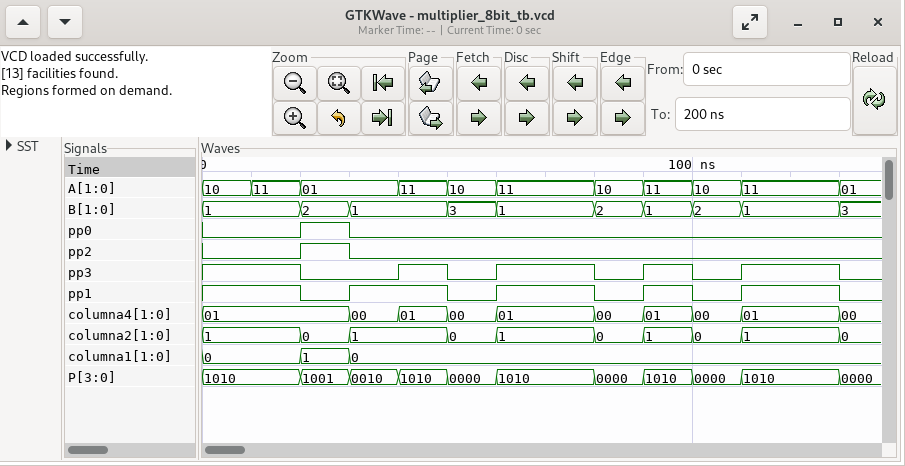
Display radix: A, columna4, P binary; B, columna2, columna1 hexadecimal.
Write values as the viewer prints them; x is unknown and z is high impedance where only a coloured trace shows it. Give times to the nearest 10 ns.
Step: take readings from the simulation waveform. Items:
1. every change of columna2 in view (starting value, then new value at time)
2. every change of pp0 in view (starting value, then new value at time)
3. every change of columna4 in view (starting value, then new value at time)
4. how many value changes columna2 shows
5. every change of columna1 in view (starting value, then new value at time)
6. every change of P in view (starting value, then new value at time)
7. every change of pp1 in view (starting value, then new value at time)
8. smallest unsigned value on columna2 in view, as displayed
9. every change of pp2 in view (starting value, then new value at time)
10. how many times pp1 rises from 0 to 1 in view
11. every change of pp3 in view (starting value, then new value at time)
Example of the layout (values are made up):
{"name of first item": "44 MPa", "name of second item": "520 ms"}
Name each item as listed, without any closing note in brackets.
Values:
{"every change of columna2 in view": "1, 0 at 20 ns, 1 at 30 ns, 0 at 50 ns, 1 at 60 ns, 0 at 80 ns, 1 at 90 ns, 0 at 100 ns, 1 at 110 ns, 0 at 130 ns", "every change of pp0 in view": "0, 1 at 20 ns, 0 at 30 ns", "every change of columna4 in view": "01, 00 at 30 ns, 01 at 40 ns, 00 at 50 ns, 01 at 60 ns, 00 at 80 ns, 01 at 90 ns, 00 at 100 ns, 01 at 110 ns, 00 at 130 ns", "how many value changes columna2 shows": "9", "every change of columna1 in view": "0, 1 at 20 ns, 0 at 30 ns", "every change of P in view": "1010, 1001 at 20 ns, 0010 at 30 ns, 1010 at 40 ns, 0000 at 50 ns, 1010 at 60 ns, 0000 at 80 ns, 1010 at 90 ns, 0000 at 100 ns, 1010 at 110 ns, 0000 at 130 ns", "every change of pp1 in view": "1, 0 at 20 ns, 1 at 30 ns, 0 at 50 ns, 1 at 60 ns, 0 at 80 ns, 1 at 90 ns, 0 at 100 ns, 1 at 110 ns, 0 at 130 ns", "smallest unsigned value on columna2 in view, as displayed": "0", "every change of pp2 in view": "0, 1 at 20 ns, 0 at 30 ns", "how many times pp1 rises from 0 to 1 in view": "4", "every change of pp3 in view": "1, 0 at 20 ns, 1 at 40 ns, 0 at 50 ns, 1 at 60 ns, 0 at 80 ns, 1 at 90 ns, 0 at 100 ns, 1 at 110 ns, 0 at 130 ns"}
